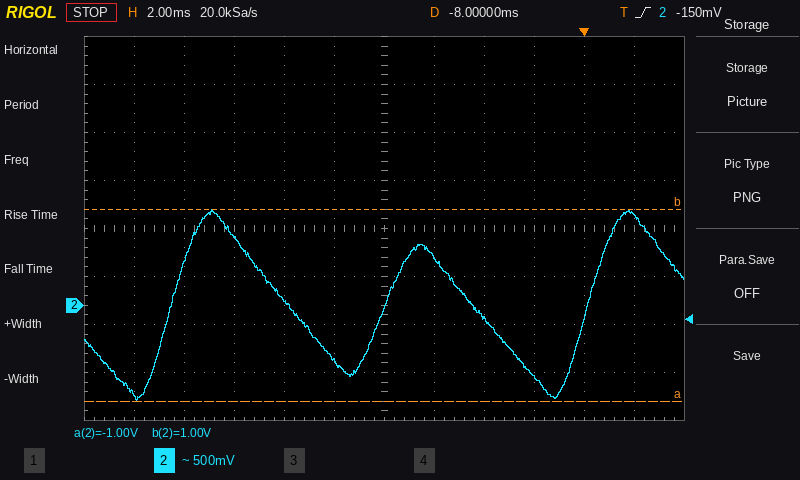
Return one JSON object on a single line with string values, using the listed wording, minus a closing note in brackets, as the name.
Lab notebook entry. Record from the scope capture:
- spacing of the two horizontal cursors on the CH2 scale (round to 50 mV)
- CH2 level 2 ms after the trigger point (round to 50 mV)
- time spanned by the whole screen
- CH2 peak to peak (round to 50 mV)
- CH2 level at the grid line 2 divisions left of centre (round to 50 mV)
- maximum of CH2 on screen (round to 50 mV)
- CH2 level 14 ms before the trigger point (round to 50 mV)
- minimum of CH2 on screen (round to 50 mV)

{"spacing of the two horizontal cursors on the CH2 scale": "2.00 V", "CH2 level 2 ms after the trigger point": "950 mV", "time spanned by the whole screen": "24 ms", "CH2 peak to peak": "2.00 V", "CH2 level at the grid line 2 divisions left of centre": "50 mV", "maximum of CH2 on screen": "1.00 V", "CH2 level 14 ms before the trigger point": "700 mV", "minimum of CH2 on screen": "-1.00 V"}
